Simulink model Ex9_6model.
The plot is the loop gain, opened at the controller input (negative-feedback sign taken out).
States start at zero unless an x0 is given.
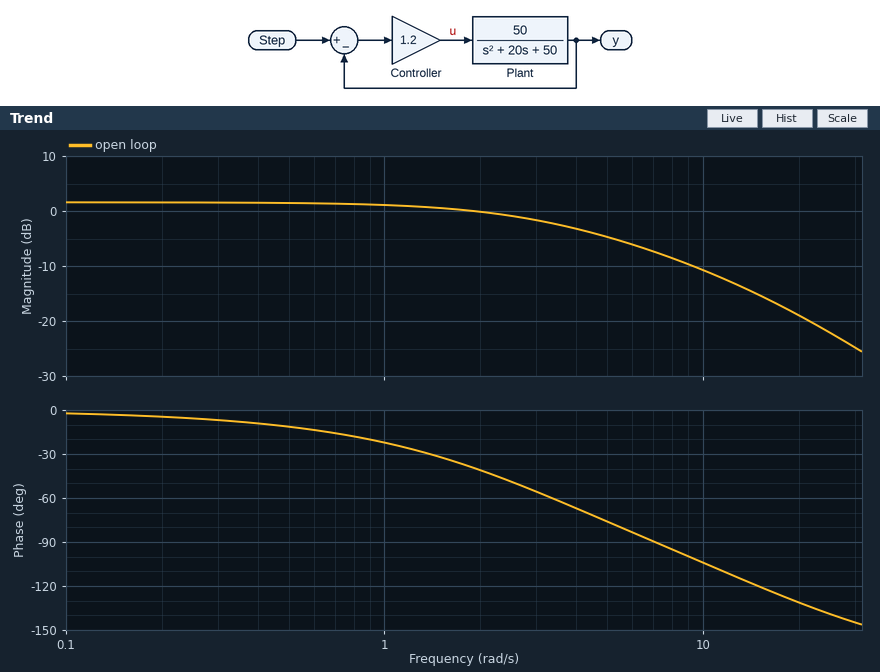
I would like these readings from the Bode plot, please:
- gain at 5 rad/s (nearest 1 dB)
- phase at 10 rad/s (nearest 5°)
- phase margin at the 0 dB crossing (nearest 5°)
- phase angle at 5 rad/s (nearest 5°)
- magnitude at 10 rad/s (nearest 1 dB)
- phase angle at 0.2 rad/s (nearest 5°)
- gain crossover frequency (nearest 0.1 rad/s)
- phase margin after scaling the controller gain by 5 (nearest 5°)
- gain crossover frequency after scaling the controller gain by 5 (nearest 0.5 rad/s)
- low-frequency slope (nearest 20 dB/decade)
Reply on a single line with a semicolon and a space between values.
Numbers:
-5 dB; -105°; 140°; -75°; -11 dB; -5°; 1.9 rad/s; 65°; 13.5 rad/s; 0 dB/decade
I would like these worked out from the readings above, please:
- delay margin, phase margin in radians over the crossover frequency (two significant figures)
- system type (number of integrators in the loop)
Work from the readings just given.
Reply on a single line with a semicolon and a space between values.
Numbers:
1.3 s; 0
